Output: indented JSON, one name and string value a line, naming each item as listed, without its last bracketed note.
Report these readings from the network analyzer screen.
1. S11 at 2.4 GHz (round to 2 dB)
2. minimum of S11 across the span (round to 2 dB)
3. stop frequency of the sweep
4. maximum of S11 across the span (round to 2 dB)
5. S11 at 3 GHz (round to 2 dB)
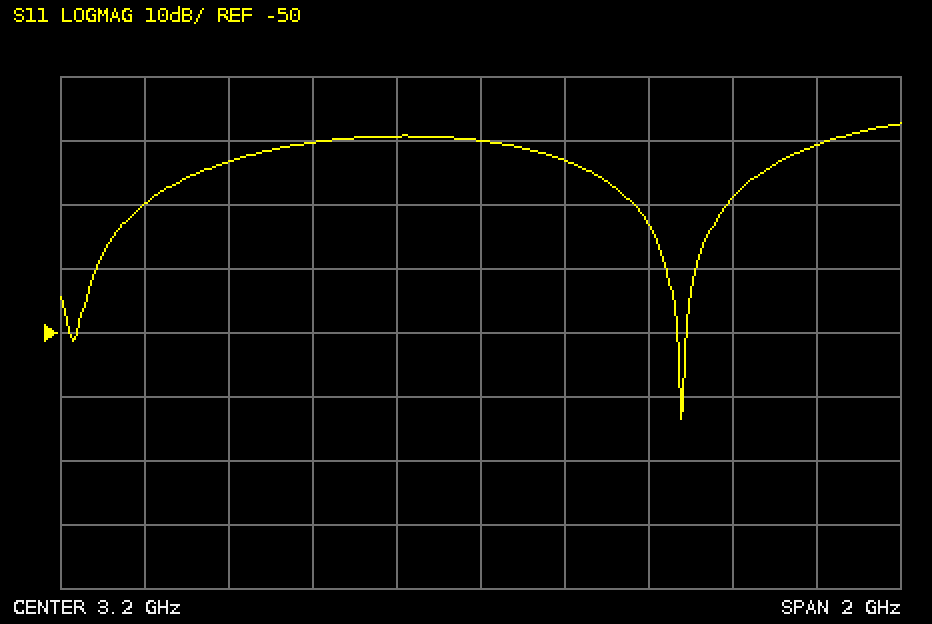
{
  "S11 at 2.4 GHz": "-30 dB",
  "minimum of S11 across the span": "-64 dB",
  "stop frequency of the sweep": "4.2 GHz",
  "maximum of S11 across the span": "-18 dB",
  "S11 at 3 GHz": "-20 dB"
}
